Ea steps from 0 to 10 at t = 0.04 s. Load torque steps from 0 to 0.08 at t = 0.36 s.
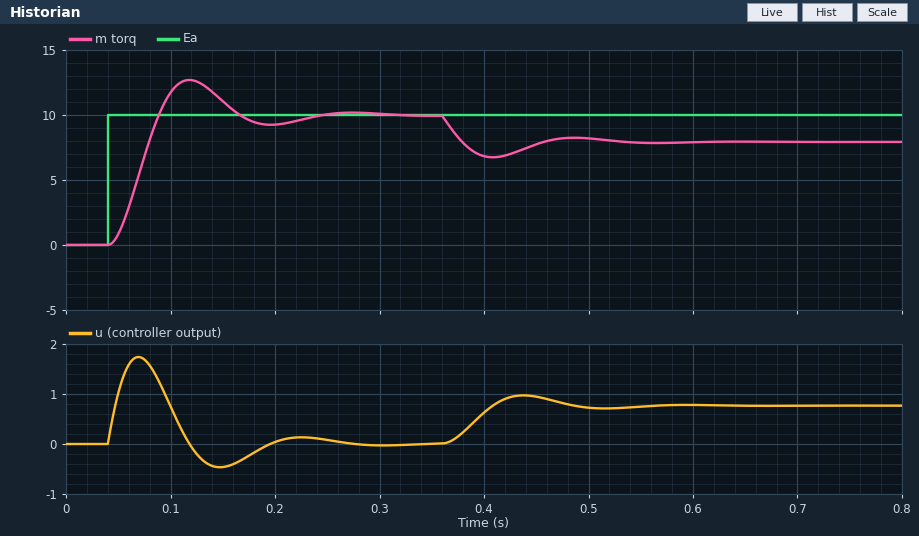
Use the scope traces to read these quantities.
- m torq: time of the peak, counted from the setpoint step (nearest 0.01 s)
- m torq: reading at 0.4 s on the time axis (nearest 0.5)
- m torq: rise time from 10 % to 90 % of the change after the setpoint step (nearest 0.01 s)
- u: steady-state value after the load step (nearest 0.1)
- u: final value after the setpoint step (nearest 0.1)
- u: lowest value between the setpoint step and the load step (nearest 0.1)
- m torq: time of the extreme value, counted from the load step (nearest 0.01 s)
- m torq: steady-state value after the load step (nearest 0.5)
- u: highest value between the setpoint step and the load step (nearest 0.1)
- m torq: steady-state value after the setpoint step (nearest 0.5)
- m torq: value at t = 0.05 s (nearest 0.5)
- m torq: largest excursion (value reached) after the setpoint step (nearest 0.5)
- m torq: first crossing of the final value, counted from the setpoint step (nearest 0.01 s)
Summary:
0.08 s
7.0
0.03 s
0.8
0.0
-0.5
0.05 s
8.0
1.7
10.0
1.0
12.5
0.05 s
